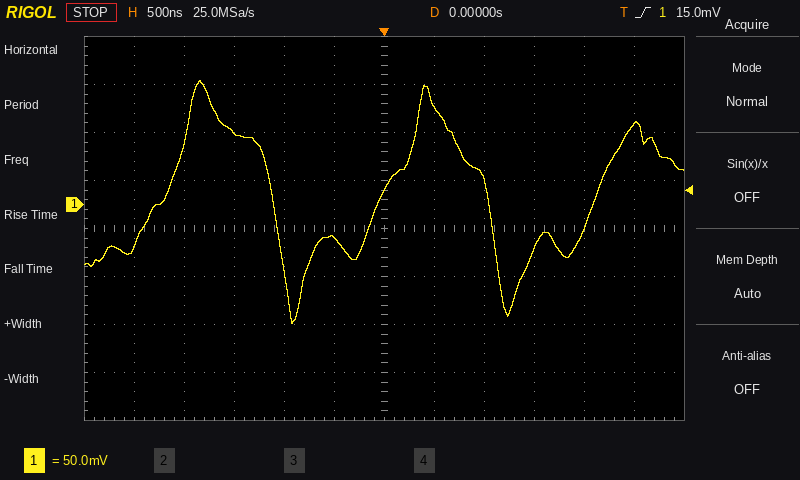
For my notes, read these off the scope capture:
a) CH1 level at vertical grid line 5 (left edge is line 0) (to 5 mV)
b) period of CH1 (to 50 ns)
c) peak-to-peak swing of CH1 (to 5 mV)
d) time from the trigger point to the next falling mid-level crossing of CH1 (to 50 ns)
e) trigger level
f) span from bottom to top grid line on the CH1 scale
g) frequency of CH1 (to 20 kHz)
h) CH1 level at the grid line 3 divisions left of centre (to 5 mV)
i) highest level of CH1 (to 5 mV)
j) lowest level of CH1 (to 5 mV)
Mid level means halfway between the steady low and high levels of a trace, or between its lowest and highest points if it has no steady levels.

-35 mV
2.15 µs
255 mV
1.05 µs
15.0 mV
400 mV
460 kHz
75 mV
130 mV
-125 mV
